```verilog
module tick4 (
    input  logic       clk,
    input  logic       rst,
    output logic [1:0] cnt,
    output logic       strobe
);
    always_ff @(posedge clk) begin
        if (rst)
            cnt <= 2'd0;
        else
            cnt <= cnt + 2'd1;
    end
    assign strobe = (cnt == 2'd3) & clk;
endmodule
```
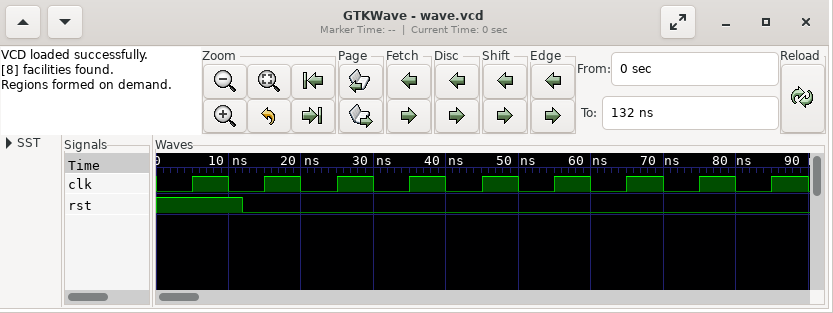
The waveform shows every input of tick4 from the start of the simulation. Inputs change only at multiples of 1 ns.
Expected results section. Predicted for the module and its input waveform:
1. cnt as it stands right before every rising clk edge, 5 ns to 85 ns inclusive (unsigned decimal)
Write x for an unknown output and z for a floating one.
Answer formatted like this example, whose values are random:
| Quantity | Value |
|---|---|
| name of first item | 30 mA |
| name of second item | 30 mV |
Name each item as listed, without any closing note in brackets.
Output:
| Quantity | Value |
|---|---|
| cnt as it stands right before every rising clk edge, 5 ns to 85 ns inclusive | x, 0, 1, 2, 3, 0, 1, 2, 3 |
